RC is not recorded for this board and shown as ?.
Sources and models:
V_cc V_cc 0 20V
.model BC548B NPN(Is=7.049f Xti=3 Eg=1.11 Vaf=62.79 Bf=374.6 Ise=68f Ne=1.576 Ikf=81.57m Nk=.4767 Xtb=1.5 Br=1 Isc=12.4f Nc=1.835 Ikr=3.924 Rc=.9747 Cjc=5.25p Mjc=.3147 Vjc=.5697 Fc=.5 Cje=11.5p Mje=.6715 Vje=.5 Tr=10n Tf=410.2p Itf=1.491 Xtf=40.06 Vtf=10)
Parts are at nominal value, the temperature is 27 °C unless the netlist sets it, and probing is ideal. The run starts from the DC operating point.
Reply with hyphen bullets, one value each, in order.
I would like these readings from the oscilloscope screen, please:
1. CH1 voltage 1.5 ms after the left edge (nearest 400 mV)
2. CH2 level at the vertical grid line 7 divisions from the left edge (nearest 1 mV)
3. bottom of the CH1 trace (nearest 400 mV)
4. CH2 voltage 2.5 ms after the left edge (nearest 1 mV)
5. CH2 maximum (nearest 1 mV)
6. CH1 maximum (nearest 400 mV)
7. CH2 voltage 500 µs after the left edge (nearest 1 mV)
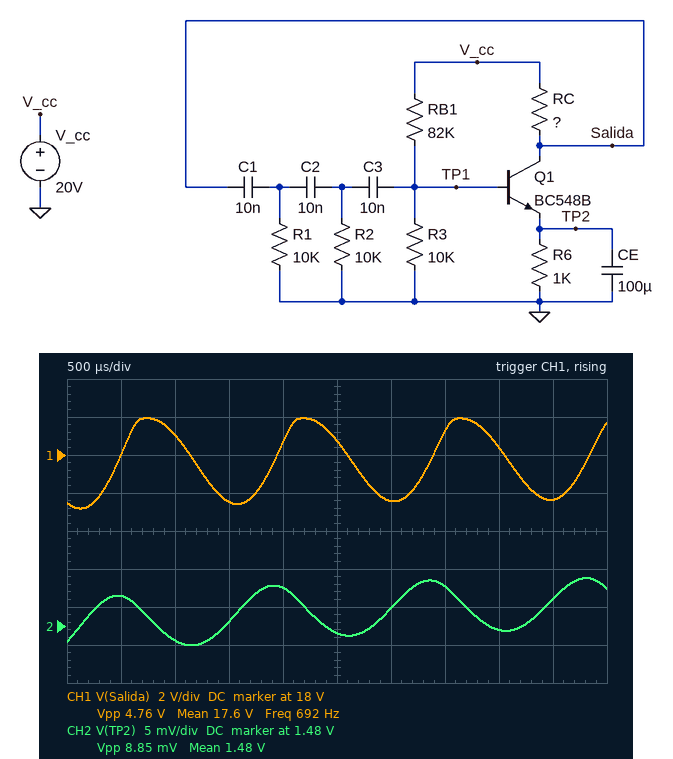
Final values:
- 15.6 V
- 1.485 V
- 15.2 V
- 1.479 V
- 1.486 V
- 20.0 V
- 1.484 V
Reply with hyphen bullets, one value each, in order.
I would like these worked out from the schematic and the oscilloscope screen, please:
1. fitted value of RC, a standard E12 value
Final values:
- 1.5 kΩ
